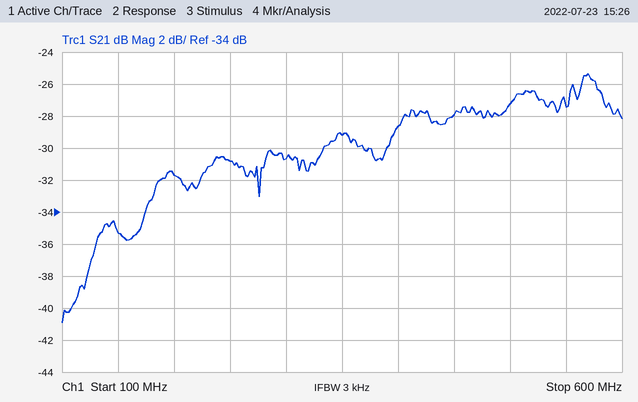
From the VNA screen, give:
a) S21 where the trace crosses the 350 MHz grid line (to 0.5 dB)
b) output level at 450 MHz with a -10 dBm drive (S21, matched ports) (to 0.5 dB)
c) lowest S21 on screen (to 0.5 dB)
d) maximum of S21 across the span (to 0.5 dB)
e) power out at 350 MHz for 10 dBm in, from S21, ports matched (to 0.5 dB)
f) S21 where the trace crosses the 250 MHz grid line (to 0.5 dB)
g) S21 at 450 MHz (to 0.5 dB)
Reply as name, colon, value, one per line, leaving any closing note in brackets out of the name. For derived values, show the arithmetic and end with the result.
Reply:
S21 where the trace crosses the 350 MHz grid line: -29.0 dB
output level at 450 MHz with a -10 dBm drive (S21, matched ports): -10 dBm + (-28.0 dB) = -38.0 dBm
lowest S21 on screen: -41.0 dB
maximum of S21 across the span: -25.5 dB
power out at 350 MHz for 10 dBm in, from S21, ports matched: 10 dBm + (-29.0 dB) = -19.0 dBm
S21 where the trace crosses the 250 MHz grid line: -31.0 dB
S21 at 450 MHz: -28.0 dB
